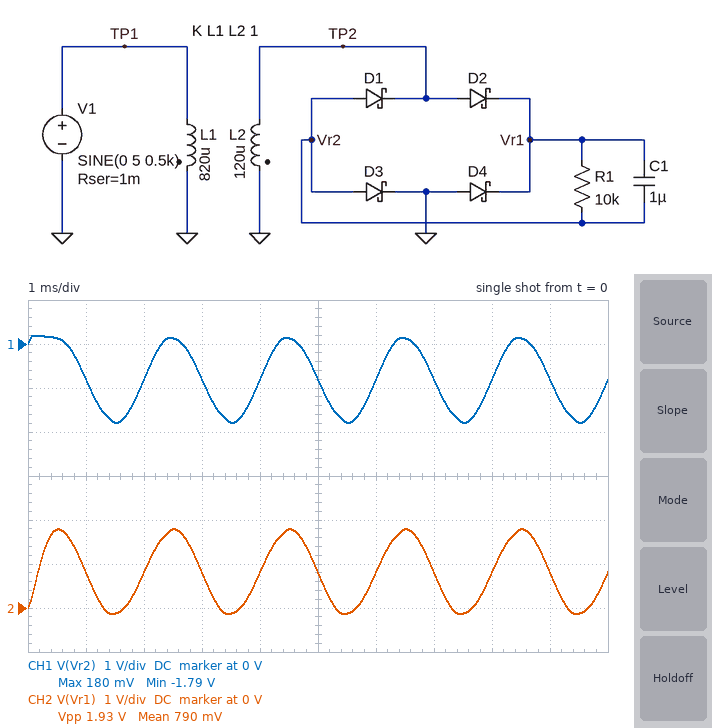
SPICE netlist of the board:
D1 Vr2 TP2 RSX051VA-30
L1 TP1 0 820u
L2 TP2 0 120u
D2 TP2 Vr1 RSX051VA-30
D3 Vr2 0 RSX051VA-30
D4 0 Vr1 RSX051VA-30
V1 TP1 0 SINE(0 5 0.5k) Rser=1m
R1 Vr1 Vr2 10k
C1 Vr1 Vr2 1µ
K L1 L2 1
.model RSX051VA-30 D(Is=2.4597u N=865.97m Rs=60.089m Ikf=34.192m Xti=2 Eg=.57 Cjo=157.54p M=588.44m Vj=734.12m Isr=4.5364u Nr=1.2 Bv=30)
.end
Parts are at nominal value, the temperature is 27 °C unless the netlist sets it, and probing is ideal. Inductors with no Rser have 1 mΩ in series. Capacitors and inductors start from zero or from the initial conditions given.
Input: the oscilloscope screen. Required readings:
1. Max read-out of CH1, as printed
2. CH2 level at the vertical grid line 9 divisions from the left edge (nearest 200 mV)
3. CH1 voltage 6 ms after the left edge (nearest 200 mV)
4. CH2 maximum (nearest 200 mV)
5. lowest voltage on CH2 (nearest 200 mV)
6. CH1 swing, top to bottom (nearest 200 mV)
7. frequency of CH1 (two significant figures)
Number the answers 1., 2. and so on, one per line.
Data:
1. 180 mV
2. 800 mV
3. -800 mV
4. 1.8 V
5. -200 mV
6. 2.0 V
7. 500 Hz
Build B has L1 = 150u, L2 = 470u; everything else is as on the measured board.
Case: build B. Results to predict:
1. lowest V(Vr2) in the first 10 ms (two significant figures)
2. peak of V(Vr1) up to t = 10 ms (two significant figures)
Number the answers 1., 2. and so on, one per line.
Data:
1. -8.7 V
2. 8.7 V
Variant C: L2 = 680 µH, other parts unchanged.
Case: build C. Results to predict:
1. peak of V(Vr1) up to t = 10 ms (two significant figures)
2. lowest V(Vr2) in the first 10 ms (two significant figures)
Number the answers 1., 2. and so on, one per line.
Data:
1. 4.4 V
2. -4.4 V
